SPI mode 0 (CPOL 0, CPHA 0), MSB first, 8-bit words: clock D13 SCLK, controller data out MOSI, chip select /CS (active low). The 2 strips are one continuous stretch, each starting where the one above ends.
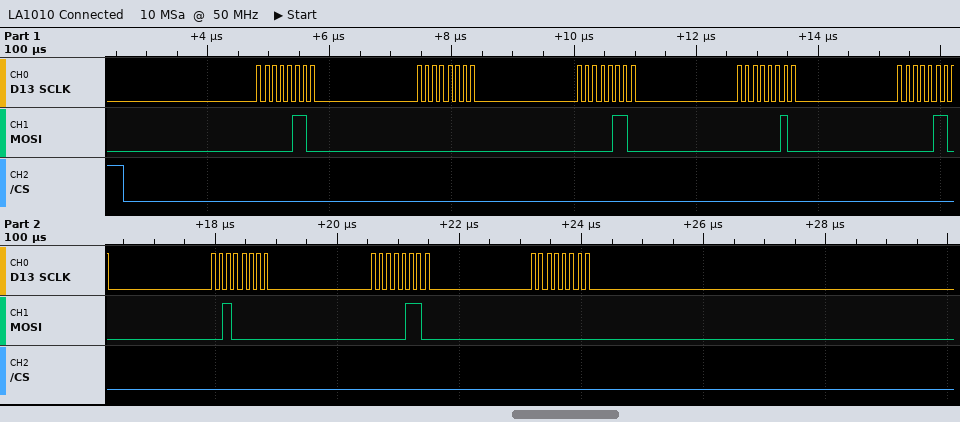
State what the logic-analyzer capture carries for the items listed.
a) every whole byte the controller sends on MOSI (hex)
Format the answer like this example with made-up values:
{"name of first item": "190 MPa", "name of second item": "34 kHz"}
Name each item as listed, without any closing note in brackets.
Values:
{"every whole byte the controller sends on MOSI": "0x06 0x00 0x06 0x02 0x06 0x20 0x06 0x00"}
